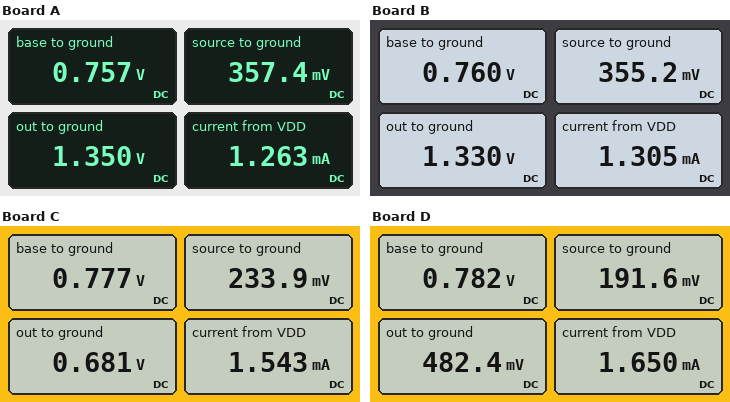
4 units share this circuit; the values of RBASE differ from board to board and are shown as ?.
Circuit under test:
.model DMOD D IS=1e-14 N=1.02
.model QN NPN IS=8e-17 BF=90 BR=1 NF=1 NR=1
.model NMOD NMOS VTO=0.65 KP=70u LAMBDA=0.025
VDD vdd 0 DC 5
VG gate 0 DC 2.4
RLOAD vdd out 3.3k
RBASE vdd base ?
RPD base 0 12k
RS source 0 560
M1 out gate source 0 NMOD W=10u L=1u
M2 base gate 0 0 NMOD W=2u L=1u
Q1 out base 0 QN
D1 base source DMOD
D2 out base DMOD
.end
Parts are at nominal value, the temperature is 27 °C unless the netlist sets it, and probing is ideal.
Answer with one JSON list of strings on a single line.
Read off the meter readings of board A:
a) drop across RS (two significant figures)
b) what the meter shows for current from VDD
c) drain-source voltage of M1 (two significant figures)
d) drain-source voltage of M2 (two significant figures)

["360 mV", "1.263 mA", "990 mV", "760 mV"]
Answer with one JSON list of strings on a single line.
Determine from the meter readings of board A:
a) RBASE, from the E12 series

["27 kΩ"]
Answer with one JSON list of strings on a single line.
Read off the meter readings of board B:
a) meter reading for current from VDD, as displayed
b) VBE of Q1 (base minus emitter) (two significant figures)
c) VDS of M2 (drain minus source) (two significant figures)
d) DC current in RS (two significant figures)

["1.305 mA", "760 mV", "760 mV", "630 µA"]
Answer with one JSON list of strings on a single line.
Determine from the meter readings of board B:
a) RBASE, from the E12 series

["22 kΩ"]
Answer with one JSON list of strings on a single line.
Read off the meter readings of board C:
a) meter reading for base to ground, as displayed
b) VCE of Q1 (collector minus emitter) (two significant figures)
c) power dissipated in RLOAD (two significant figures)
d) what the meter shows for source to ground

["0.777 V", "680 mV", "5.7 mW", "233.9 mV"]
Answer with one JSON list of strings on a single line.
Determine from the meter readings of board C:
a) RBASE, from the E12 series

["18 kΩ"]
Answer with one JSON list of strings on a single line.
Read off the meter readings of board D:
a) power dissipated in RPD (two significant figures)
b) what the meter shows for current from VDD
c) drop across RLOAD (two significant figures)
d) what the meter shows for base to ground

["51 µW", "1.650 mA", "4.5 V", "0.782 V"]
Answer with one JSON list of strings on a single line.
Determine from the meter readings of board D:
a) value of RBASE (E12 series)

["15 kΩ"]
